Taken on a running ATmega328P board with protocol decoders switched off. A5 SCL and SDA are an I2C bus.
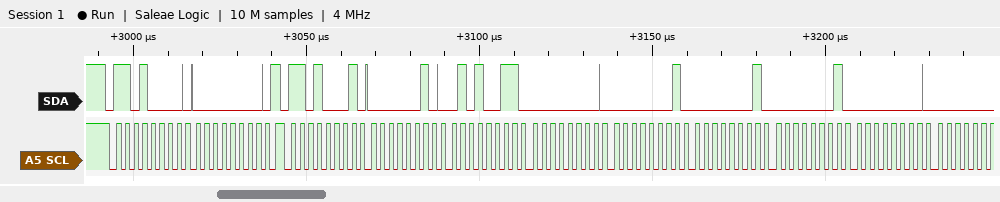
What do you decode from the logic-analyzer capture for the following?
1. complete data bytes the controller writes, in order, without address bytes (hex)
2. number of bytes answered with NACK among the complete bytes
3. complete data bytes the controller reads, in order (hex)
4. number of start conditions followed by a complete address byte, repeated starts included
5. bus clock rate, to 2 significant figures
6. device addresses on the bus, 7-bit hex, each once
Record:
00
0
02 53 00 01 01 01 00
2
400 kHz
0x68
